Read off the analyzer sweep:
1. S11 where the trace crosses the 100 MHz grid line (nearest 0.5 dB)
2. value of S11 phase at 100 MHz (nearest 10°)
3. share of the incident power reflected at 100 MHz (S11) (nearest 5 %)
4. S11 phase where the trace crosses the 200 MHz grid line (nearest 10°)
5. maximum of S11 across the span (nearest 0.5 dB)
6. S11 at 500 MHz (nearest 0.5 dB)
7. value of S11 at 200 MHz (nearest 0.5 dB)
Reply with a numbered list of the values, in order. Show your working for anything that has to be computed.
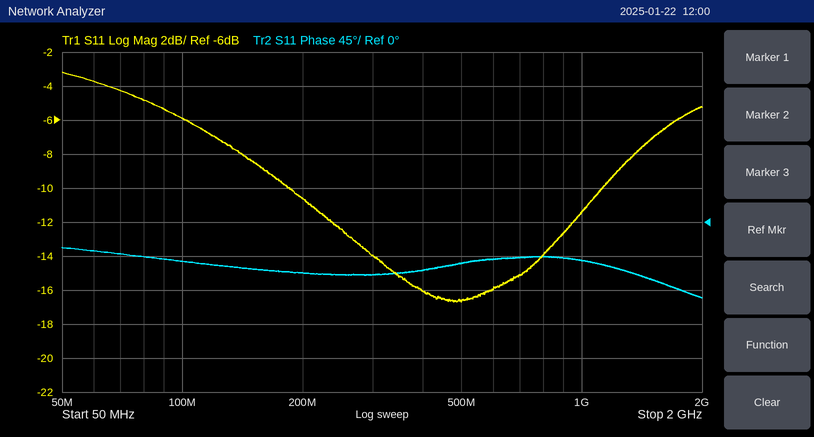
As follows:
1. -6.0 dB
2. -50°
3. 10^(-6/10) ≈ 25 %
4. -70°
5. -3.0 dB
6. -16.5 dB
7. -10.5 dB
